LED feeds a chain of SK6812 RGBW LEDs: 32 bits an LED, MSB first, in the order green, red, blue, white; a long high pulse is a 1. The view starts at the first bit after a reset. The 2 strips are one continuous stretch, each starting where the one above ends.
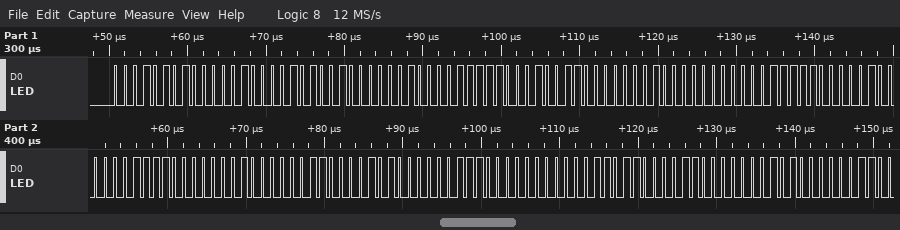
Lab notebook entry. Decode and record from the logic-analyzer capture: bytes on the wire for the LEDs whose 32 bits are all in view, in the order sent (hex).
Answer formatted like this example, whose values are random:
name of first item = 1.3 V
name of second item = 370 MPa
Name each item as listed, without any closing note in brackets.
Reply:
bytes on the wire for the LEDs whose 32 bits are all in view, in the order sent = 15 04 29 02 1F 13 01 00 1F 04 0F 01 03 0A 07 00 1B 0C 05 03
